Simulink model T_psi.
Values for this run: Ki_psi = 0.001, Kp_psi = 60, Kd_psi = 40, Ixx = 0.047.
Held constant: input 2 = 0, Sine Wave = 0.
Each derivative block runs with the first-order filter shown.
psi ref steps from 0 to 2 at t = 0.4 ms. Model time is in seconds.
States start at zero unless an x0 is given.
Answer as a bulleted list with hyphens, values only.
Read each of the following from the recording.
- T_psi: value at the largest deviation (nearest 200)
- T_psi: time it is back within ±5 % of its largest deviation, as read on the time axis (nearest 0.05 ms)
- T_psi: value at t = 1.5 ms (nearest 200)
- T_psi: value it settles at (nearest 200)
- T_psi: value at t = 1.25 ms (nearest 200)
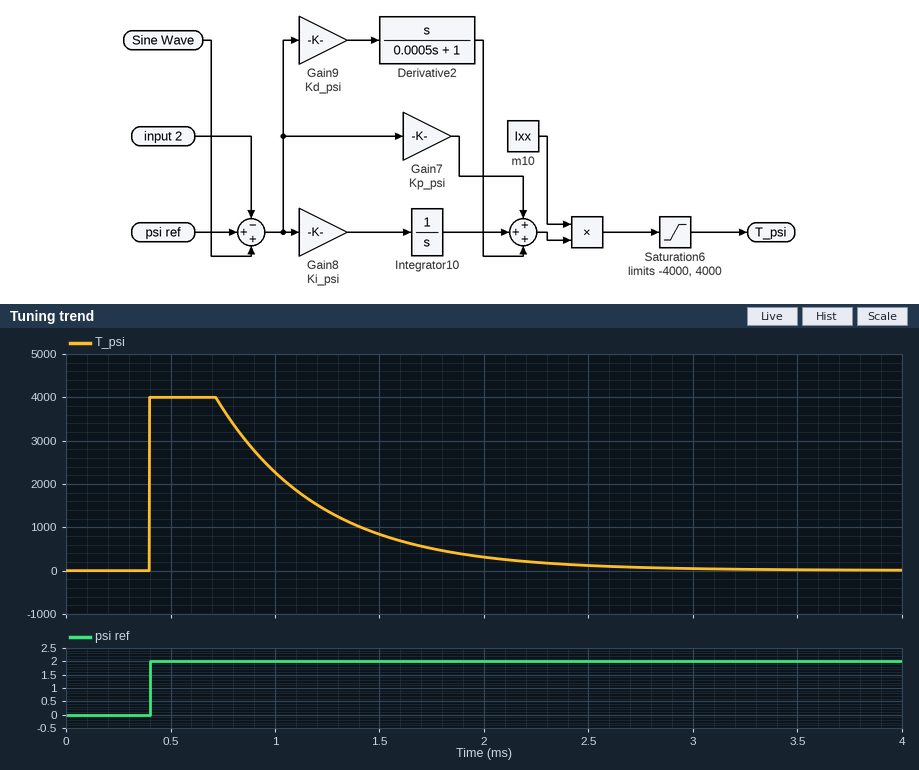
- 4000
- 2.20 ms
- 800
- 0
- 1400
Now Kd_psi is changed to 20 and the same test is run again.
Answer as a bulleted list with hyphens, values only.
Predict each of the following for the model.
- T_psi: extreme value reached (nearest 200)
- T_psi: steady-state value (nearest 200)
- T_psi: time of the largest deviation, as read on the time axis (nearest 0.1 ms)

- 3800
- 0
- 0.4 ms
